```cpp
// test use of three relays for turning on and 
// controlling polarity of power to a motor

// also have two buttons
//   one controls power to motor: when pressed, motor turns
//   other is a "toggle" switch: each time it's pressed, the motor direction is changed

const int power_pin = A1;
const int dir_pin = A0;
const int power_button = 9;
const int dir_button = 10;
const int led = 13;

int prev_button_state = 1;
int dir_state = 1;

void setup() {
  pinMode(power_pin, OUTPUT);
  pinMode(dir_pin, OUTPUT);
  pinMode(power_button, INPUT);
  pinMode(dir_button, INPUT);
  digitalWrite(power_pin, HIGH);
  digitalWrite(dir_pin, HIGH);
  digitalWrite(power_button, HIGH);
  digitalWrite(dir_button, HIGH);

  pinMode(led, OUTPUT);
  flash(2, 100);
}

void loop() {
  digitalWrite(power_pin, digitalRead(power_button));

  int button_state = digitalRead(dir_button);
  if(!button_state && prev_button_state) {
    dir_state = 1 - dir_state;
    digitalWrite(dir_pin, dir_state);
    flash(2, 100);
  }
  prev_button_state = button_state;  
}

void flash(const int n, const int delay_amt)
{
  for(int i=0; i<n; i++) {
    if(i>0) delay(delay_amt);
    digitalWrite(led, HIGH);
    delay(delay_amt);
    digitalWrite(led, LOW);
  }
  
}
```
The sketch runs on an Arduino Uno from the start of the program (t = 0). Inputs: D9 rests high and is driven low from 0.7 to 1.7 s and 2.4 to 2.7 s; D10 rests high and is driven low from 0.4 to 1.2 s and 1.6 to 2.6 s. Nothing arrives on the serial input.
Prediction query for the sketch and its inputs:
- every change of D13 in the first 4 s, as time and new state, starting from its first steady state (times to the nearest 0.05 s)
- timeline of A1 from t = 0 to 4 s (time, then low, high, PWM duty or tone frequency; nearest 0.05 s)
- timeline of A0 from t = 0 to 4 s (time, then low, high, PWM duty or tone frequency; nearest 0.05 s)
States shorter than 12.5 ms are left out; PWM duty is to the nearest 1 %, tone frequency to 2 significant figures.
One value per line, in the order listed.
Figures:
0 s high; 0.1 s low; 0.2 s high; 0.3 s low; 0.4 s high; 0.5 s low; 0.6 s high; 0.7 s low; 1.6 s high; 1.7 s low; 1.8 s high; 1.9 s low
0 s high; 0.7 s low; 1.9 s high; 2.4 s low; 2.7 s high
0 s high; 0.4 s low; 1.6 s high
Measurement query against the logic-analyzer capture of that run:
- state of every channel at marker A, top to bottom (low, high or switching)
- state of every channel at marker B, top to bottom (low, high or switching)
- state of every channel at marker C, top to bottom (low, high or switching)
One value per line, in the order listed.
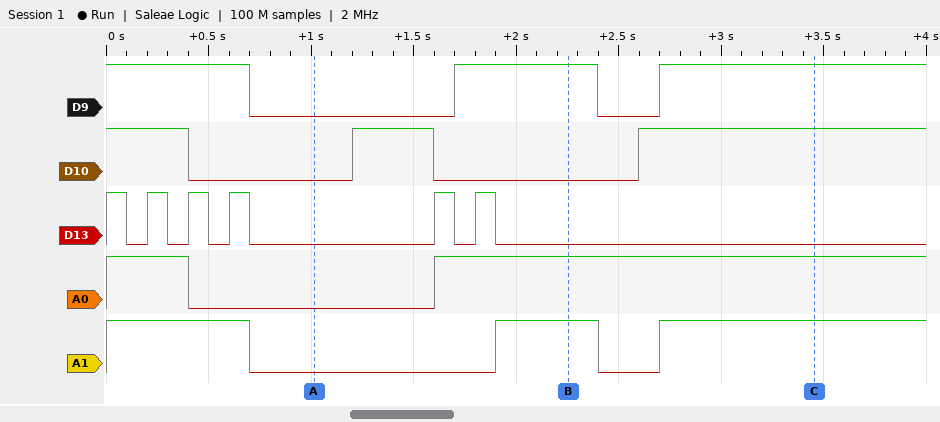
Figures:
D9 low, D10 low, D13 low, A0 low, A1 low
D9 high, D10 low, D13 low, A0 high, A1 high
D9 high, D10 high, D13 low, A0 high, A1 high
